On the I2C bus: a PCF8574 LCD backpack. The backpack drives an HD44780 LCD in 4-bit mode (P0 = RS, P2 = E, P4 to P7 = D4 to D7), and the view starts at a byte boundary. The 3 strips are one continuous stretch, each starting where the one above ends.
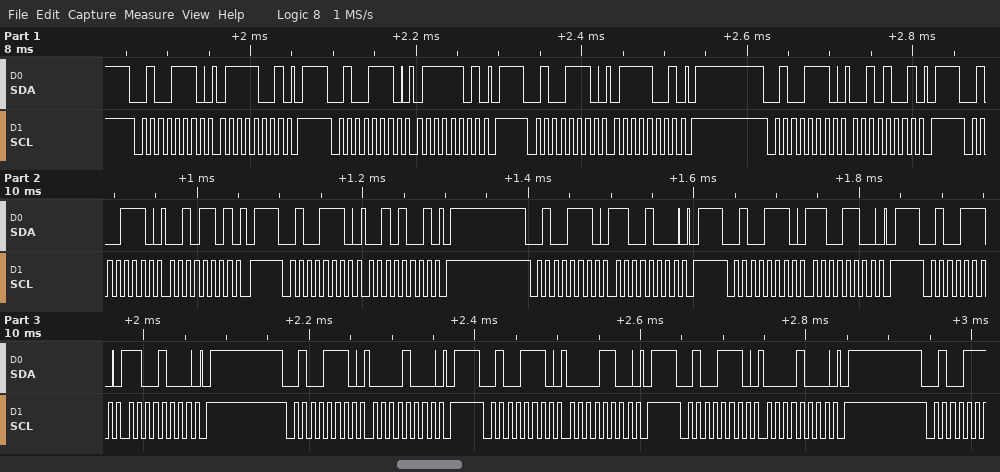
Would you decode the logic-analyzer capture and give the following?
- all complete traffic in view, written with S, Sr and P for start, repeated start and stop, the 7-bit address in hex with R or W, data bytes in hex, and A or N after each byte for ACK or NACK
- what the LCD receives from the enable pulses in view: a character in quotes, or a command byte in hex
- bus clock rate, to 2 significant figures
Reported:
S 27W A 79 A P S 27W A 7D A P S 27W A 79 A P S 27W A 29 A P S 27W A 2D A P S 27W A 29 A P S 27W A C8 A P S 27W A CC A P S 27W A C8 A P S 27W A 08 A P S 27W A 0C A P S 27W A 08 A P
'r' 0xC0
100 kHz
